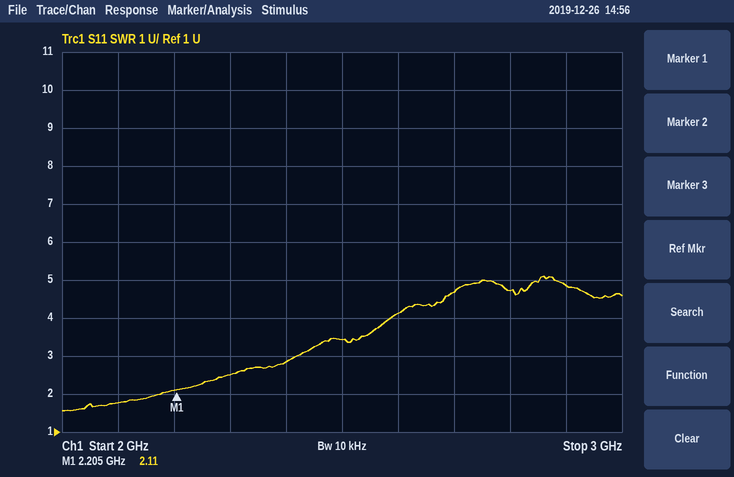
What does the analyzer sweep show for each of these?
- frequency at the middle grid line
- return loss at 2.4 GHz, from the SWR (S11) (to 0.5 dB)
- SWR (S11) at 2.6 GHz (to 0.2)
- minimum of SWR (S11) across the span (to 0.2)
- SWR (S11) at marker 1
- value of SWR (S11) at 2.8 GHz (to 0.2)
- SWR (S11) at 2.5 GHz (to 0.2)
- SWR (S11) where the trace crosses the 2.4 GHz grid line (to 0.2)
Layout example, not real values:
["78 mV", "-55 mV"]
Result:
["2.5 GHz", "6.5 dB", "4.2", "1.6", "2.11", "4.8", "3.4", "2.8"]
